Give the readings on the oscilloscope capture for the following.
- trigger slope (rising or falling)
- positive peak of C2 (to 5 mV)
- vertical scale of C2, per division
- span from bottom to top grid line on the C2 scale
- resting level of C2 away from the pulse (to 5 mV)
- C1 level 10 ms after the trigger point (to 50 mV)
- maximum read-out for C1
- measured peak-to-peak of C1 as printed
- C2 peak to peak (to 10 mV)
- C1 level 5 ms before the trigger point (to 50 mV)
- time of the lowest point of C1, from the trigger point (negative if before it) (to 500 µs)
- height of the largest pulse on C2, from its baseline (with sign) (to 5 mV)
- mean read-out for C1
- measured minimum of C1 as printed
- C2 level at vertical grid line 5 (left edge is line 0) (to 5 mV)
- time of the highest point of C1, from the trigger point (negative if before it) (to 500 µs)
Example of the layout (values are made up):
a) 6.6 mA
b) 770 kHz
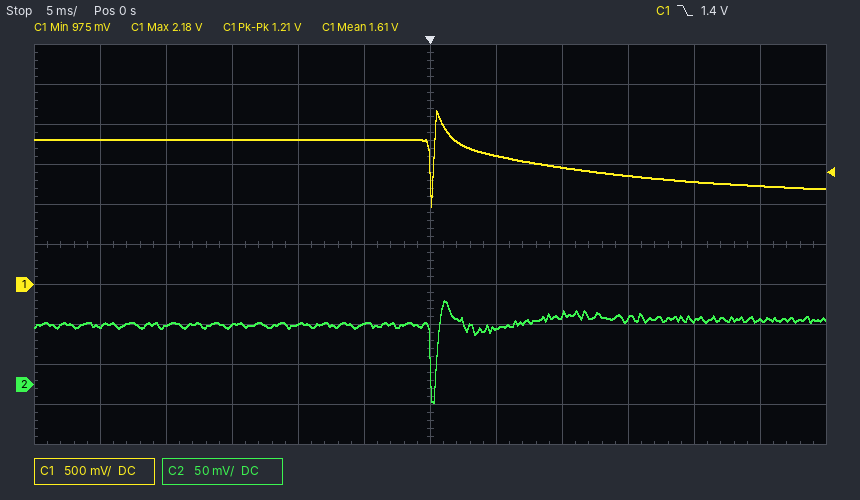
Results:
a) falling
b) 105 mV
c) 50 mV
d) 500 mV
e) 75 mV
f) 1.45 V
g) 2.18 V
h) 1.21 V
i) 130 mV
j) 1.80 V
k) 0.0 ms
l) -100 mV
m) 1.61 V
n) 975 mV
o) 75 mV
p) +500 µs
